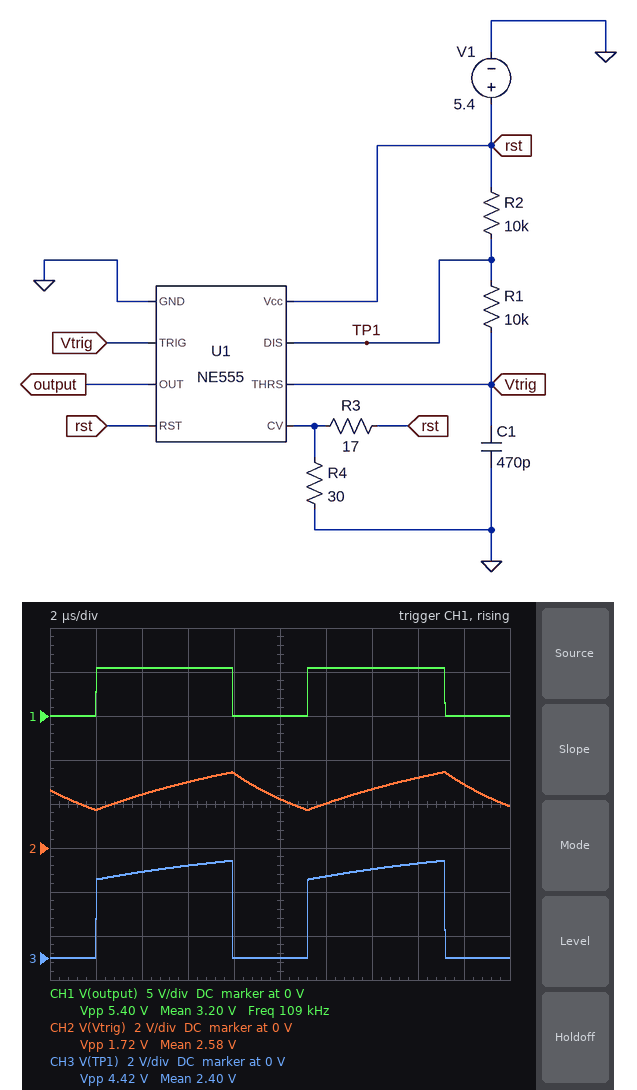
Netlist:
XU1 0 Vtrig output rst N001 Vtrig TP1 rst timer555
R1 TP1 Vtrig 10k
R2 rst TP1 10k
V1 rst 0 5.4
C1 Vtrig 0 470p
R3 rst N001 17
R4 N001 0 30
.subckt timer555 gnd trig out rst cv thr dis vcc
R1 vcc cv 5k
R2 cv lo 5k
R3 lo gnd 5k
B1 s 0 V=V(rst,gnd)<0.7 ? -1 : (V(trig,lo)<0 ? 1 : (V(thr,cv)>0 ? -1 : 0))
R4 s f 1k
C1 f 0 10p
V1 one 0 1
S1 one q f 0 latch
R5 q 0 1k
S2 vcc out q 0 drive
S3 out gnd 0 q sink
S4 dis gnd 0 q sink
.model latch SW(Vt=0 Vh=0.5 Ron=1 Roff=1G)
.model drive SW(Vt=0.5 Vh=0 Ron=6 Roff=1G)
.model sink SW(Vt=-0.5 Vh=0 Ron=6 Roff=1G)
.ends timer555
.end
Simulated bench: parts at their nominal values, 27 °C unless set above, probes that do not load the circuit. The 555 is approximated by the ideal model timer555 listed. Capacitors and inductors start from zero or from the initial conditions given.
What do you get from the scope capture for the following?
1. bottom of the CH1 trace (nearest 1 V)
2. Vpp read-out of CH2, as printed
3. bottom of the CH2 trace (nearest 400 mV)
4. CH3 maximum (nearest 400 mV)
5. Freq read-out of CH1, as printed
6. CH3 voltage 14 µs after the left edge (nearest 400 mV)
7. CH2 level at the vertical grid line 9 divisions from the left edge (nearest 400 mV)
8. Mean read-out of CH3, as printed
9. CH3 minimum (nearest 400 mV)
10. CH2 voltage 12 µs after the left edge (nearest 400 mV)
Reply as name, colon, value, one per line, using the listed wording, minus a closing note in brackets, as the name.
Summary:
bottom of the CH1 trace: 0 V
Vpp read-out of CH2, as printed: 1.72 V
bottom of the CH2 trace: 1.6 V
CH3 maximum: 4.4 V
Freq read-out of CH1, as printed: 109 kHz
CH3 voltage 14 µs after the left edge: 4.0 V
CH2 level at the vertical grid line 9 divisions from the left edge: 2.8 V
Mean read-out of CH3, as printed: 2.40 V
CH3 minimum: 0 V
CH2 voltage 12 µs after the left edge: 2.0 V
